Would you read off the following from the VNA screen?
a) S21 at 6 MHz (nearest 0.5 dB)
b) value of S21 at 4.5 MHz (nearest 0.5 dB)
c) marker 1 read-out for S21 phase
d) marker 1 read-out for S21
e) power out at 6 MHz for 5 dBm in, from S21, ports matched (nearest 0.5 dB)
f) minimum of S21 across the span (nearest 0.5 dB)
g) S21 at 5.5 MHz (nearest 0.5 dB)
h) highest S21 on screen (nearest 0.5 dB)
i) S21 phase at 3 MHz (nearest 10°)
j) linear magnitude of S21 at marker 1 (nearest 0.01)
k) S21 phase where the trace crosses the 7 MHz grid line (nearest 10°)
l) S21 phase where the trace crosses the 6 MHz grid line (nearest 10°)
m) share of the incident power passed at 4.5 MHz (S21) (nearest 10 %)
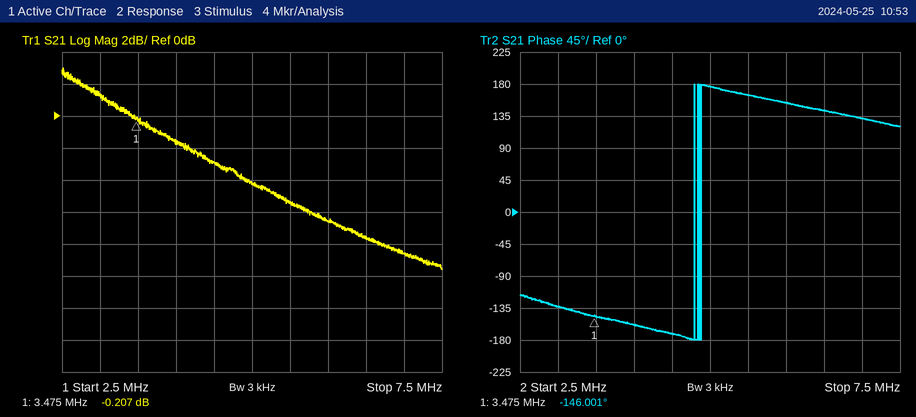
-6.5 dB
-3.0 dB
-146.001°
-0.207 dB
-1.5 dBm
-9.5 dB
-5.5 dB
3.0 dB
-130°
0.98
130°
150°
50 %
